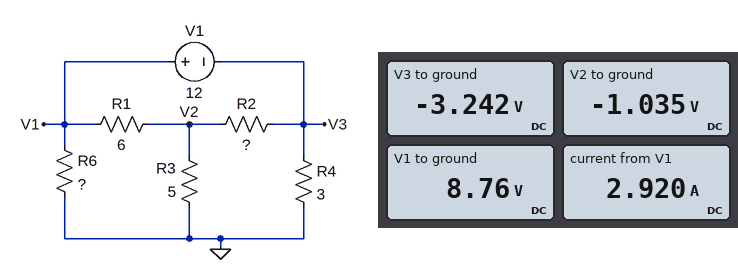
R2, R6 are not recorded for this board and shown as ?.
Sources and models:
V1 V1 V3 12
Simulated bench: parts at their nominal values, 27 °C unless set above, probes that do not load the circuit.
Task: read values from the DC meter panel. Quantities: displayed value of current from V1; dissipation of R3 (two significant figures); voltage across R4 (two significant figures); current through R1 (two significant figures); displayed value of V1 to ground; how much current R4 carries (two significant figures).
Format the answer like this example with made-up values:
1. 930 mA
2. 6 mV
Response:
1. 2.920 A
2. 210 mW
3. 3.2 V
4. 1.6 A
5. 8.76 V
6. 1.1 A
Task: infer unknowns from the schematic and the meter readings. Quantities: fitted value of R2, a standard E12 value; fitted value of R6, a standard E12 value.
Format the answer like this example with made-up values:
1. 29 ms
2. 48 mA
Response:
1. 1.2 Ω
2. 6.8 Ω
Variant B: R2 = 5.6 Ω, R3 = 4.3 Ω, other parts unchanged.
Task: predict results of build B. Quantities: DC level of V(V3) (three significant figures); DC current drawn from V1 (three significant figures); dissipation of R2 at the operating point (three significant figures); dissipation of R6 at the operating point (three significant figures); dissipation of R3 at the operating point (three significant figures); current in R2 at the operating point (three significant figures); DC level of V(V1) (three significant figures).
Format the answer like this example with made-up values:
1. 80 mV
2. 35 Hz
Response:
1. -4.15 V
2. 2.30 A
3. 4.70 W
4. 9.06 W
5. 224 mW
6. 916 mA
7. 7.85 V
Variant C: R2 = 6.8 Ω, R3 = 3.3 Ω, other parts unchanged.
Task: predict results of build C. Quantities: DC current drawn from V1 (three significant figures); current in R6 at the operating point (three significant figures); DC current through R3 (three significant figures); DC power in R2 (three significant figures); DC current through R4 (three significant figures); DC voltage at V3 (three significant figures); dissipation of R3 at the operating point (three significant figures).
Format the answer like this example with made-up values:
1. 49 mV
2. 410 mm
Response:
1. 2.23 A
2. 1.13 A
3. 315 mA
4. 4.24 W
5. 1.44 A
6. -4.33 V
7. 328 mW
